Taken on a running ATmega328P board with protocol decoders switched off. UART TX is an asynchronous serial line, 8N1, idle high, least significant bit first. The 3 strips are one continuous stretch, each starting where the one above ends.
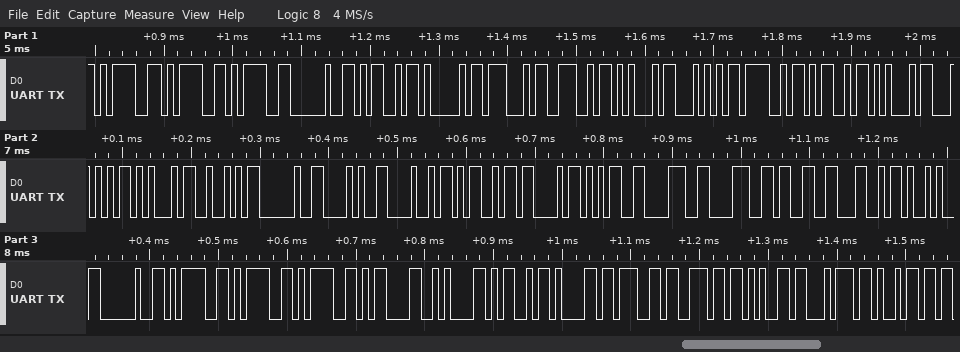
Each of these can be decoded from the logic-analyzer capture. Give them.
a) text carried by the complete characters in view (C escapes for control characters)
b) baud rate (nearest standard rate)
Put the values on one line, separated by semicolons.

"=== MAGNETOMETER (HMC5883L) ===\r\nMagneti"; 115200 baud
